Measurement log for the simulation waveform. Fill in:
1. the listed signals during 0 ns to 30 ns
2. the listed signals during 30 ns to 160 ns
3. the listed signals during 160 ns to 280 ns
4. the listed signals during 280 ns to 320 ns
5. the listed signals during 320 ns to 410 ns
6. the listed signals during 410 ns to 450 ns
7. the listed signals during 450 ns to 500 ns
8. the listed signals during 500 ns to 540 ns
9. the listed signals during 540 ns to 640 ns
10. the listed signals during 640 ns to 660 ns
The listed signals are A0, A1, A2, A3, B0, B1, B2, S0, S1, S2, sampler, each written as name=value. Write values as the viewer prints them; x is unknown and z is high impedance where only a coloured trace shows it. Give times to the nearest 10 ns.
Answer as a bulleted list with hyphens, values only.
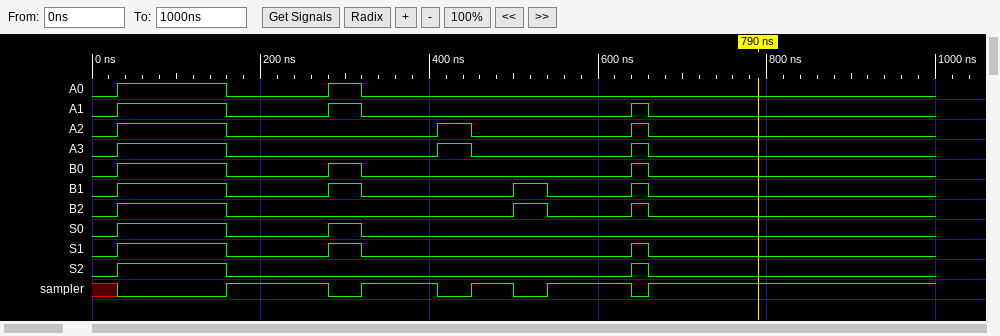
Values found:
- A0=0, A1=0, A2=0, A3=0, B0=0, B1=0, B2=0, S0=0, S1=0, S2=0, sampler=x
- A0=1, A1=1, A2=1, A3=1, B0=1, B1=1, B2=1, S0=1, S1=1, S2=1, sampler=0
- A0=0, A1=0, A2=0, A3=0, B0=0, B1=0, B2=0, S0=0, S1=0, S2=0, sampler=1
- A0=1, A1=1, A2=0, A3=0, B0=1, B1=1, B2=0, S0=1, S1=1, S2=0, sampler=0
- A0=0, A1=0, A2=0, A3=0, B0=0, B1=0, B2=0, S0=0, S1=0, S2=0, sampler=1
- A0=0, A1=0, A2=1, A3=1, B0=0, B1=0, B2=0, S0=0, S1=0, S2=0, sampler=0
- A0=0, A1=0, A2=0, A3=0, B0=0, B1=0, B2=0, S0=0, S1=0, S2=0, sampler=1
- A0=0, A1=0, A2=0, A3=0, B0=0, B1=1, B2=1, S0=0, S1=0, S2=0, sampler=0
- A0=0, A1=0, A2=0, A3=0, B0=0, B1=0, B2=0, S0=0, S1=0, S2=0, sampler=1
- A0=0, A1=1, A2=1, A3=1, B0=1, B1=1, B2=1, S0=0, S1=1, S2=1, sampler=0
